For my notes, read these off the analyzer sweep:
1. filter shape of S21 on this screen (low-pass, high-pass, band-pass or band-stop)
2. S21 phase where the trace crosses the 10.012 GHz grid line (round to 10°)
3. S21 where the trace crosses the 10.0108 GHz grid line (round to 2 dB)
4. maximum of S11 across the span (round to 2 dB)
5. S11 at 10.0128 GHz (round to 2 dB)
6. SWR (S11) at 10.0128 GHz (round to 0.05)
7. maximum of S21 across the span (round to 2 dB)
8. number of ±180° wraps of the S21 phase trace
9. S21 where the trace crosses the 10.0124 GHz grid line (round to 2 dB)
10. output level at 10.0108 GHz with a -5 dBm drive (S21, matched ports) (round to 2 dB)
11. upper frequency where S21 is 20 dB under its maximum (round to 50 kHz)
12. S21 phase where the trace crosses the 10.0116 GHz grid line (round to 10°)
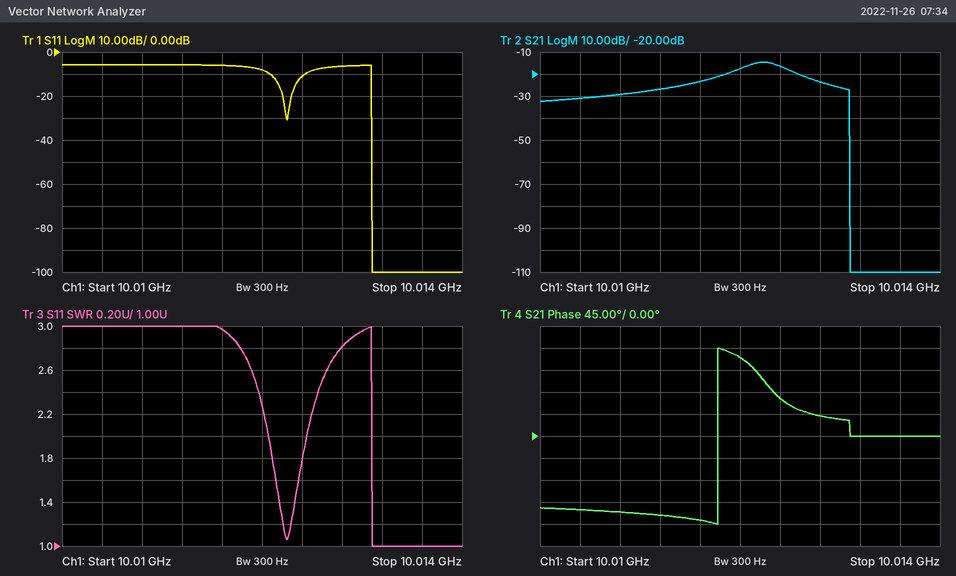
band-pass
160°
-30 dB
-6 dB
-6 dB
2.80
-14 dB
1
-16 dB
-34 dBm
10.01310 GHz
-170°
